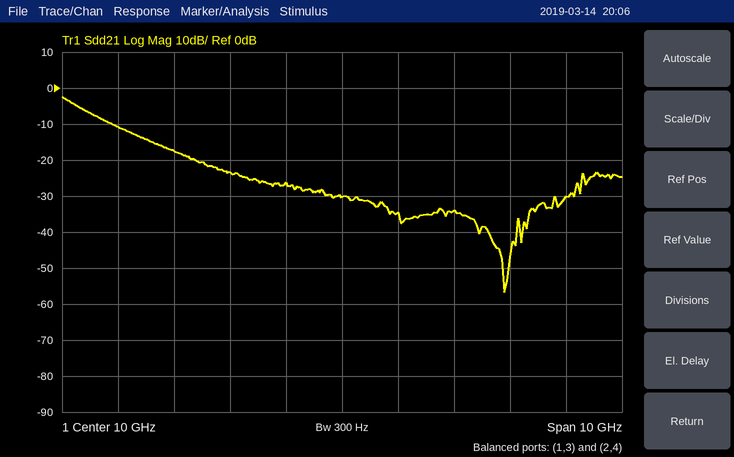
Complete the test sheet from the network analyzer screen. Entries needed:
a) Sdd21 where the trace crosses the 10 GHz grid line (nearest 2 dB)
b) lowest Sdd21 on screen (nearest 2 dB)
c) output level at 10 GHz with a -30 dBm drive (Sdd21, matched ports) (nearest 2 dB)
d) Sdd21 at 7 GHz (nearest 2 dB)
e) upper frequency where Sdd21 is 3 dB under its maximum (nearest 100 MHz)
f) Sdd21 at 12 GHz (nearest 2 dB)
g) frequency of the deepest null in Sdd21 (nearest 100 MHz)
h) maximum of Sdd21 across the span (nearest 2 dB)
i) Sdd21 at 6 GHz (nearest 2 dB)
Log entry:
-30 dB
-56 dB
-60 dBm
-18 dB
5.3 GHz
-34 dB
12.9 GHz
-2 dB
-10 dB
